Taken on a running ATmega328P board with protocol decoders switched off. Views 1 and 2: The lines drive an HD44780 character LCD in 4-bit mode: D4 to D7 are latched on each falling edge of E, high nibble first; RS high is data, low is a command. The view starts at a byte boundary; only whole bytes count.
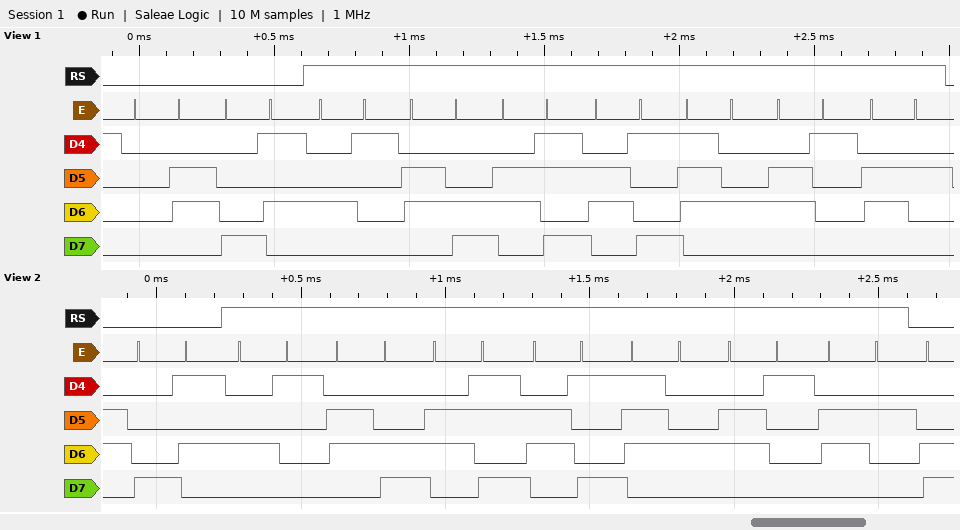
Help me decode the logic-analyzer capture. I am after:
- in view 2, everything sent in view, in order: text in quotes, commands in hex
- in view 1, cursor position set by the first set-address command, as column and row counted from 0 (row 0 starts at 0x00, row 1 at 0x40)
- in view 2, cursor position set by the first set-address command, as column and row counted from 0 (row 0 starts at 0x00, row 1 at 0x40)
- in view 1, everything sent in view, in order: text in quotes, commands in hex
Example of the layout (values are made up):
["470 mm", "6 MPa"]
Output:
["0x85 \"Alkitab\"", "column 5, row 0", "column 5, row 0", "0x06 0x85 \"Alkitab\""]
